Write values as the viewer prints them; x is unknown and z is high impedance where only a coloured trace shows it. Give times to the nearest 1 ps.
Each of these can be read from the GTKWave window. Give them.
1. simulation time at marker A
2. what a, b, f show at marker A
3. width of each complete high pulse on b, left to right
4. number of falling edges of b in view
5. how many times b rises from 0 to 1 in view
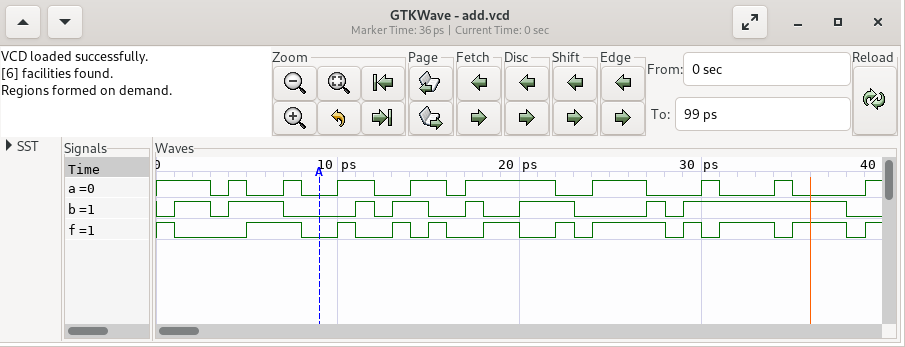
9 ps
a=0, b=0, f=0
2 ps, 3 ps, 1 ps, 2 ps, 1 ps, 3 ps, 1 ps, 9 ps
8
8
